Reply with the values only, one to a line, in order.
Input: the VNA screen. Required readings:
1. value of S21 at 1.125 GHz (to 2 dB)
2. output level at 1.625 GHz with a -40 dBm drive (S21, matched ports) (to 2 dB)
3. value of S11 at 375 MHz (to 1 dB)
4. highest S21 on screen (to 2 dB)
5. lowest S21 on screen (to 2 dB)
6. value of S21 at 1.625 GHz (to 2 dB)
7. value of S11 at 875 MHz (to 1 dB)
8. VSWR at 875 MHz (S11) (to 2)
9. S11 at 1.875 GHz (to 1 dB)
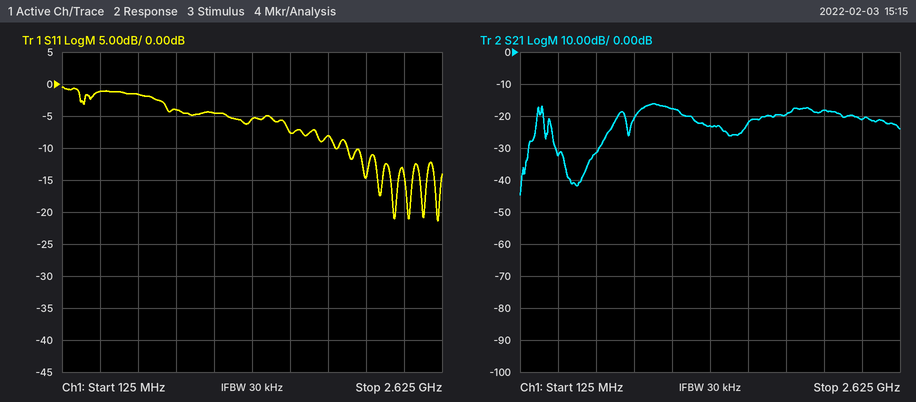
-18 dB
-62 dBm
-1 dB
-16 dB
-44 dB
-22 dB
-4 dB
4
-8 dB
